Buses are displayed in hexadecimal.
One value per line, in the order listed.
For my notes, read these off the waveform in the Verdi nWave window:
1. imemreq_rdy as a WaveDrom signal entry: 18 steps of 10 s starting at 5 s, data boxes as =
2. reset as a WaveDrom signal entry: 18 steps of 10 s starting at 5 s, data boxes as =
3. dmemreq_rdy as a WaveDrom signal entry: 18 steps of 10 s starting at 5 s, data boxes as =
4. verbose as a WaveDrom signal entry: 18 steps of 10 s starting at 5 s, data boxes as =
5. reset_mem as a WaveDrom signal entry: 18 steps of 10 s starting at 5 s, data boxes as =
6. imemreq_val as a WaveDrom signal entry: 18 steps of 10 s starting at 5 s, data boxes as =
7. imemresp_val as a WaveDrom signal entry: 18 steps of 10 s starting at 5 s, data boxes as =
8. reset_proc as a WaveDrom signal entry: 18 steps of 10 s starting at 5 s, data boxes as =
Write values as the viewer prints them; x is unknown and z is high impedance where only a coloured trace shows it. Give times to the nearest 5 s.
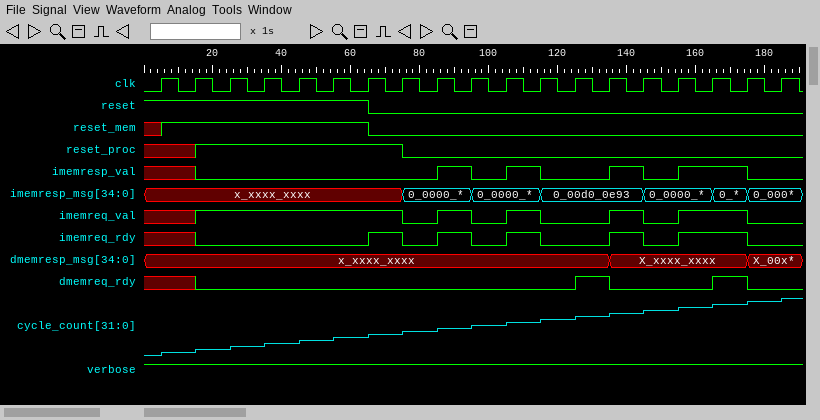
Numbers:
{name: 'imemreq_rdy', wave: 'x0....101010.101.0'}
{name: 'reset', wave: '1.....0...........'}
{name: 'dmemreq_rdy', wave: 'x0..........10..10'}
{name: 'verbose', wave: '1.................'}
{name: 'reset_mem', wave: '1.....0...........'}
{name: 'imemreq_val', wave: 'x1.....01010.101.0'}
{name: 'imemresp_val', wave: 'x0......1010.101.0'}
{name: 'reset_proc', wave: 'x1.....0..........'}
